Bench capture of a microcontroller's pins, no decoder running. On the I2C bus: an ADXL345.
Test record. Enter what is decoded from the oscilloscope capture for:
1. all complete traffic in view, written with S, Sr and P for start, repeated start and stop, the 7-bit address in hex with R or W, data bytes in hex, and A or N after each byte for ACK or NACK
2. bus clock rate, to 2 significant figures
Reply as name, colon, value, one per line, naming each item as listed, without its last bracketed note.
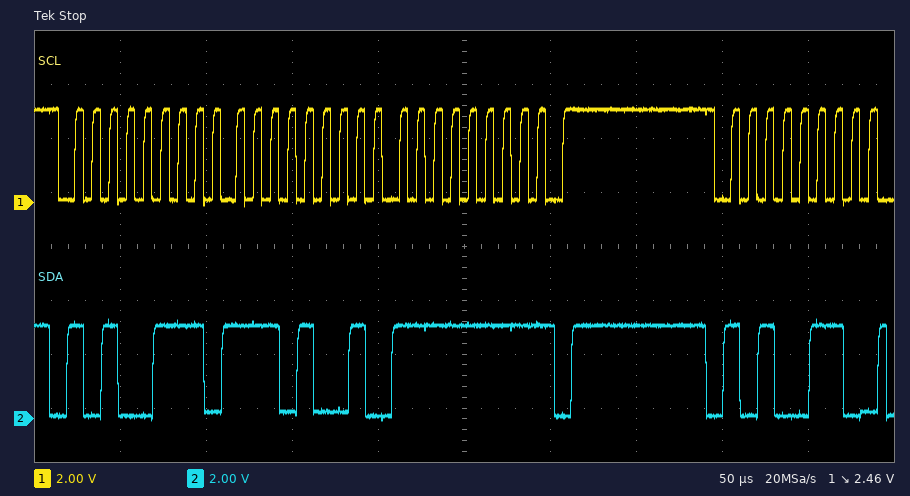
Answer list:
all complete traffic in view, written with S, Sr and P for start, repeated start and stop, the 7-bit address in hex with R or W, data bytes in hex, and A or N after each byte for ACK or NACK: S 53R A E9 A FF N P S 53W A
bus clock rate, to 2 significant figures: 100 kHz
